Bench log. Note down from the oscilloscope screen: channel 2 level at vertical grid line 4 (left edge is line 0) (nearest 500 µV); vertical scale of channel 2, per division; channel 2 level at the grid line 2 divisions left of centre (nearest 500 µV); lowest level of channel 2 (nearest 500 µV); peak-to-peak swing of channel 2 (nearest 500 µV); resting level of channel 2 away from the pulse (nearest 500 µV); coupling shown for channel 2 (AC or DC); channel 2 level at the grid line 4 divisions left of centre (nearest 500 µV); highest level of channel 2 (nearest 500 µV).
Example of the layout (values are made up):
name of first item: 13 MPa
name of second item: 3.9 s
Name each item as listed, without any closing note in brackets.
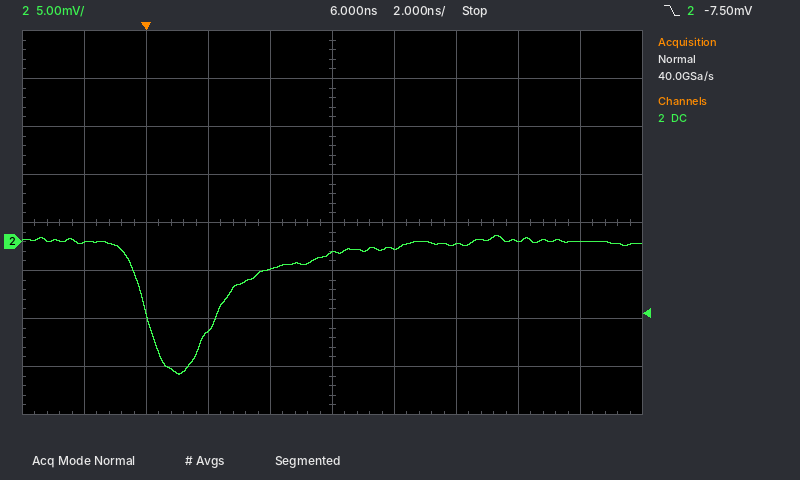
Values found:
channel 2 level at vertical grid line 4 (left edge is line 0): -3.0 mV
vertical scale of channel 2, per division: 5 mV
channel 2 level at the grid line 2 divisions left of centre: -9.5 mV
lowest level of channel 2: -14.0 mV
peak-to-peak swing of channel 2: 14.5 mV
resting level of channel 2 away from the pulse: 0.0 mV
coupling shown for channel 2: DC
channel 2 level at the grid line 4 divisions left of centre: 0.0 mV
highest level of channel 2: 500 µV
